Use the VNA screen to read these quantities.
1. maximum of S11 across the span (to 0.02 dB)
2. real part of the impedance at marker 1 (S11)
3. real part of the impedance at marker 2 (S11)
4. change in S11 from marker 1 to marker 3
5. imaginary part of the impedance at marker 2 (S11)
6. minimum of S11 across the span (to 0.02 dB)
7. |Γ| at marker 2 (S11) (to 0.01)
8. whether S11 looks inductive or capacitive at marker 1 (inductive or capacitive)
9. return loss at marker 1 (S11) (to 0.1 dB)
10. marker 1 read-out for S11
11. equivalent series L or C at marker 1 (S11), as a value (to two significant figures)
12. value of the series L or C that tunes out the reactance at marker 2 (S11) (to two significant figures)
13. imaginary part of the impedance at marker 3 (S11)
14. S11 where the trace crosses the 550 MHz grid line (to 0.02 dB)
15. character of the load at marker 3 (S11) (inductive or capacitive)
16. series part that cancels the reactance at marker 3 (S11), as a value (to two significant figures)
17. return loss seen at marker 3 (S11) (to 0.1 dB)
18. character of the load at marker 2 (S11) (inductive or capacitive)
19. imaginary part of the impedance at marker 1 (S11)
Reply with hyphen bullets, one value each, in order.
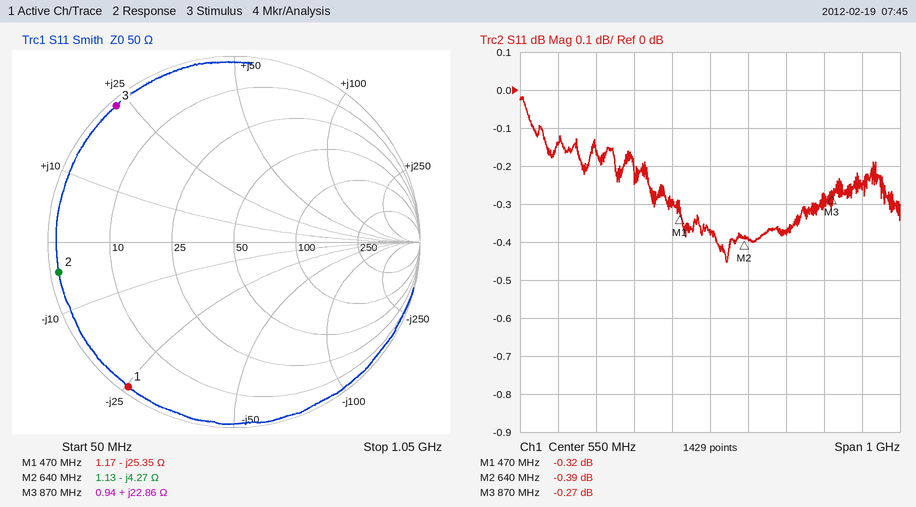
- -0.02 dB
- 1.17 Ω
- 1.13 Ω
- 0.05 dB
- -4.27 Ω
- -0.46 dB
- 0.96
- capacitive
- 0.3 dB
- -0.32 dB
- 13 pF
- 1.1 nH
- +22.86 Ω
- -0.38 dB
- inductive
- 8.0 pF
- 0.3 dB
- capacitive
- -25.35 Ω
